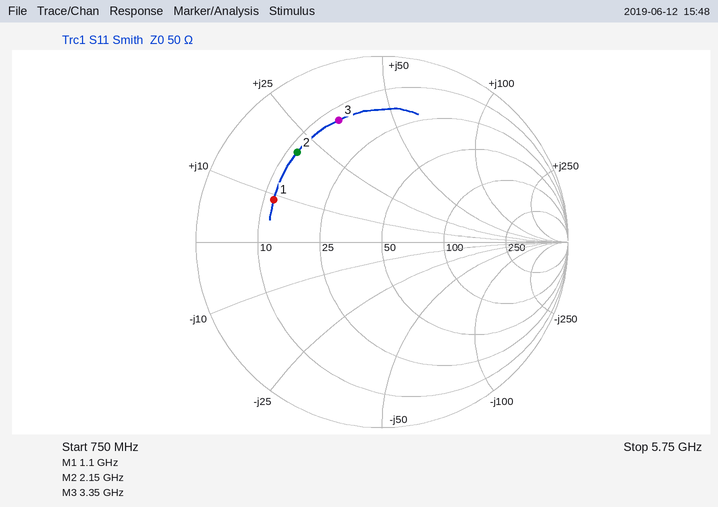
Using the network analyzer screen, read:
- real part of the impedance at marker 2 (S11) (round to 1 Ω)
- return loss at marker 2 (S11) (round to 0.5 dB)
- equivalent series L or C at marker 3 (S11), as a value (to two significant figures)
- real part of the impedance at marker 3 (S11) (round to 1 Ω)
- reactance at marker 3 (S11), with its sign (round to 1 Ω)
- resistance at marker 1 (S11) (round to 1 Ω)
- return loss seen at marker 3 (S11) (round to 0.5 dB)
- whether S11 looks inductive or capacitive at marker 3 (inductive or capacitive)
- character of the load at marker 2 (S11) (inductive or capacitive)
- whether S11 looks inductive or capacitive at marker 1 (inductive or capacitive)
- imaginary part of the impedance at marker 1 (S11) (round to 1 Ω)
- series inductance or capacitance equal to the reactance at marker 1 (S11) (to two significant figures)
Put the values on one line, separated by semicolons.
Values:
12 Ω; 3.5 dB; 1.6 nH; 13 Ω; +34 Ω; 12 Ω; 3.0 dB; inductive; inductive; inductive; +9 Ω; 1.3 nH
